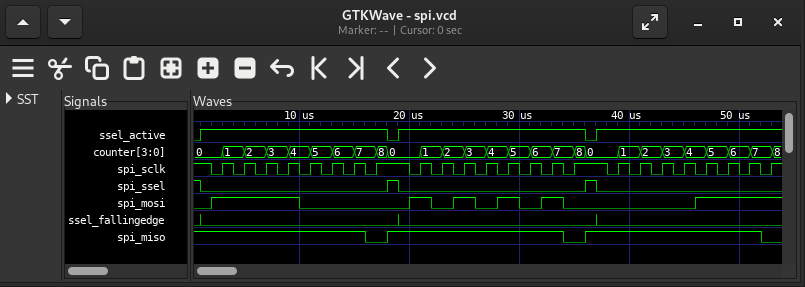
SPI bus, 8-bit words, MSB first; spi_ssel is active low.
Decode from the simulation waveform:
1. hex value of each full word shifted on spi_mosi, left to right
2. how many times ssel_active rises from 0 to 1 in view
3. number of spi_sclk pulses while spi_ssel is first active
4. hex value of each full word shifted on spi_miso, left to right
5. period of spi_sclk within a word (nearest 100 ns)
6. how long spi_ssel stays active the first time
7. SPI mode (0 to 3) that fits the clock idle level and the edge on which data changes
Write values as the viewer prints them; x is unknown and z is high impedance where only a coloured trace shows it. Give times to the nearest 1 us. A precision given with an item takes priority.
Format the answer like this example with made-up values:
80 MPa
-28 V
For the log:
F0, AA, 0F
3
8
FE, FE, FE
2000 ns
17 us
3
